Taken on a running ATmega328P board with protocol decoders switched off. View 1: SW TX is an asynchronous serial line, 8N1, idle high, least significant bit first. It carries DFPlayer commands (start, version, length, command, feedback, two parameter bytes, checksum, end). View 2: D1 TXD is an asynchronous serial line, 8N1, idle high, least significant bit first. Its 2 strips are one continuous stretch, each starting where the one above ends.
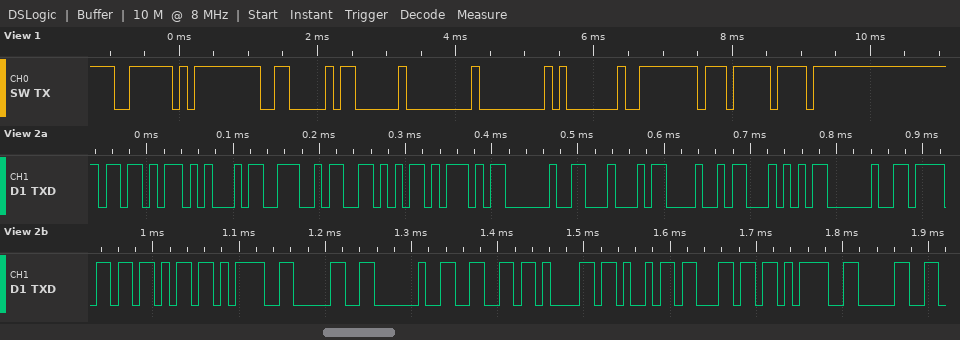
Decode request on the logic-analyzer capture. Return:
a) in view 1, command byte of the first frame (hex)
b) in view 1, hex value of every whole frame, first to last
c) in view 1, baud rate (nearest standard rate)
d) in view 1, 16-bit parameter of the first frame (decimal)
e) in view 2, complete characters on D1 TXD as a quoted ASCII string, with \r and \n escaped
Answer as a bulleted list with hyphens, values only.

- 0x03
- 0x7E 0xFF 0x06 0x03 0x00 0x00 0x01 0xFE 0xF7 0xEF
- 9600 baud
- 1
- "[ENV] DHT ok=0 fail=0"
